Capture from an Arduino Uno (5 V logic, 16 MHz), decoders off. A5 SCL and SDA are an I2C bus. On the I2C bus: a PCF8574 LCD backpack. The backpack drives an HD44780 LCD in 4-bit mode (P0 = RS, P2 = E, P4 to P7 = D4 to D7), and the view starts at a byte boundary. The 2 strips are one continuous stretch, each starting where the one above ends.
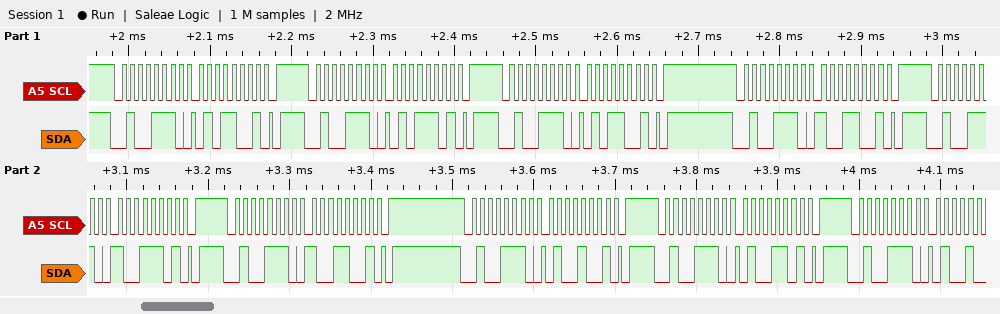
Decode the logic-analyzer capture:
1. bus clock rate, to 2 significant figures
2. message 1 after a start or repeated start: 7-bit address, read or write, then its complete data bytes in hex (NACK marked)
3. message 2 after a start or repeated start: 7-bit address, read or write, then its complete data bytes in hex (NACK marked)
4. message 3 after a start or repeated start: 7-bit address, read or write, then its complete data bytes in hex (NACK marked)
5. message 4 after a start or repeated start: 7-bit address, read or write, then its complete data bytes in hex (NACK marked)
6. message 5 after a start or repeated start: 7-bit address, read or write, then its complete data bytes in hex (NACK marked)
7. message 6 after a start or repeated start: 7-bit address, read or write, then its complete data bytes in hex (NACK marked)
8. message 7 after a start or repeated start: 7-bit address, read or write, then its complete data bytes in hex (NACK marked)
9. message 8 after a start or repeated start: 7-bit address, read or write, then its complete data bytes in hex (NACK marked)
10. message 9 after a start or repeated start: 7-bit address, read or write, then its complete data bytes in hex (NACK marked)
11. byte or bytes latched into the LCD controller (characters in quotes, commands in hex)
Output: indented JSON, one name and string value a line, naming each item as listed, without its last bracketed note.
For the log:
{
  "bus clock rate, to 2 significant figures": "100 kHz",
  "message 1 after a start or repeated start: 7-bit address, read or write, then its complete data bytes in hex": "0x27 write: 59",
  "message 2 after a start or repeated start: 7-bit address, read or write, then its complete data bytes in hex": "0x27 write: 5D",
  "message 3 after a start or repeated start: 7-bit address, read or write, then its complete data bytes in hex": "0x27 write: 59",
  "message 4 after a start or repeated start: 7-bit address, read or write, then its complete data bytes in hex": "0x27 write: 99",
  "message 5 after a start or repeated start: 7-bit address, read or write, then its complete data bytes in hex": "0x27 write: 9D",
  "message 6 after a start or repeated start: 7-bit address, read or write, then its complete data bytes in hex": "0x27 write: 99",
  "message 7 after a start or repeated start: 7-bit address, read or write, then its complete data bytes in hex": "0x27 write: 49",
  "message 8 after a start or repeated start: 7-bit address, read or write, then its complete data bytes in hex": "0x27 write: 4D",
  "message 9 after a start or repeated start: 7-bit address, read or write, then its complete data bytes in hex": "0x27 write",
  "byte or bytes latched into the LCD controller": "'Y'"
}
